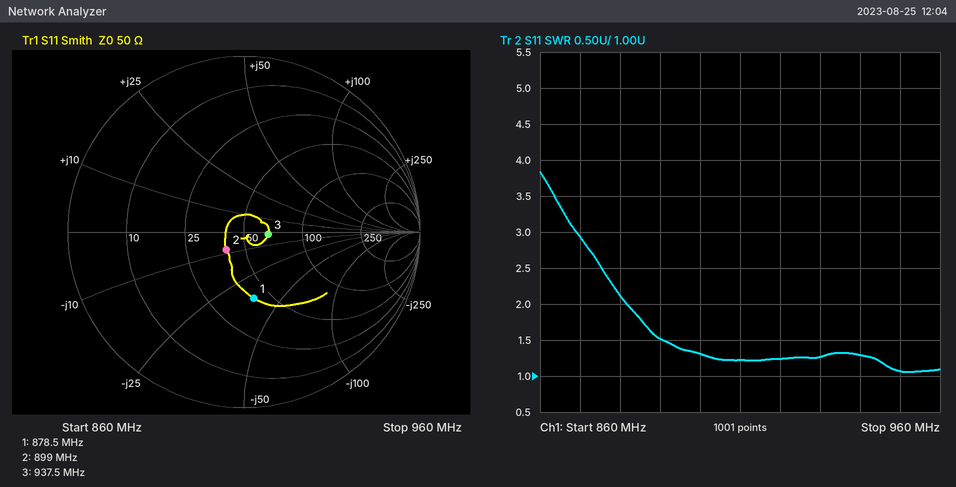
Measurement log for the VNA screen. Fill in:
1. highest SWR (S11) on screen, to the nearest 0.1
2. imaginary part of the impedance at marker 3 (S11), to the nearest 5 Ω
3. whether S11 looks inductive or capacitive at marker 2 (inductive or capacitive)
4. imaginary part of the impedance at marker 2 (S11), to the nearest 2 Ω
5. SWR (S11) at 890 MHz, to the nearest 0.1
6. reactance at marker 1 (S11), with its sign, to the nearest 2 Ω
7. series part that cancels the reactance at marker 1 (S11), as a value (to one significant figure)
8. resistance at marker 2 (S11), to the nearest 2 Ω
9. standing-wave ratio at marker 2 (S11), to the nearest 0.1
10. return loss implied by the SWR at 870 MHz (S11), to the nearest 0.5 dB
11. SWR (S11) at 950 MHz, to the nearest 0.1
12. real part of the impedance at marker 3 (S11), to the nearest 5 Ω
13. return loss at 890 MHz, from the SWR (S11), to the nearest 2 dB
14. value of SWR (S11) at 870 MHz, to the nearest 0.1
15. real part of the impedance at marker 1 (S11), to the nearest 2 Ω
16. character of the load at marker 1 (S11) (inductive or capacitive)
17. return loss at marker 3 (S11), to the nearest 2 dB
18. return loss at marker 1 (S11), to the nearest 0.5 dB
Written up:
3.8
0 Ω
capacitive
-8 Ω
1.5
-36 Ω
7 nH
40 Ω
1.3
6.0 dB
1.1
65 Ω
14 dB
2.9
42 Ω
capacitive
18 dB
8.5 dB
